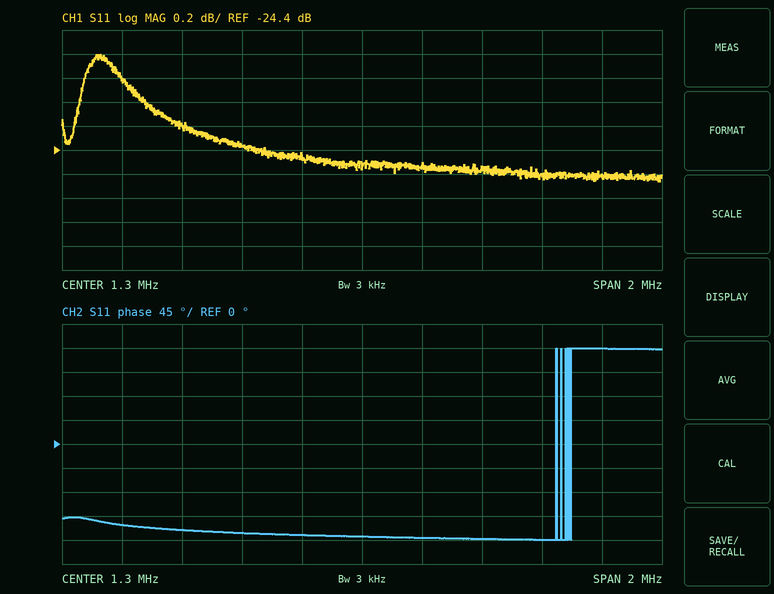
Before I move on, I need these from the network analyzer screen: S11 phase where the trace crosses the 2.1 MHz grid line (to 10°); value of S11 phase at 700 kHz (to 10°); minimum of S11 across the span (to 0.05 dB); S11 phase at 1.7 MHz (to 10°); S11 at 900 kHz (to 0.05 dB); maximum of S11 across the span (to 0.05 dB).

180°
-160°
-24.65 dB
-180°
-24.35 dB
-23.60 dB
